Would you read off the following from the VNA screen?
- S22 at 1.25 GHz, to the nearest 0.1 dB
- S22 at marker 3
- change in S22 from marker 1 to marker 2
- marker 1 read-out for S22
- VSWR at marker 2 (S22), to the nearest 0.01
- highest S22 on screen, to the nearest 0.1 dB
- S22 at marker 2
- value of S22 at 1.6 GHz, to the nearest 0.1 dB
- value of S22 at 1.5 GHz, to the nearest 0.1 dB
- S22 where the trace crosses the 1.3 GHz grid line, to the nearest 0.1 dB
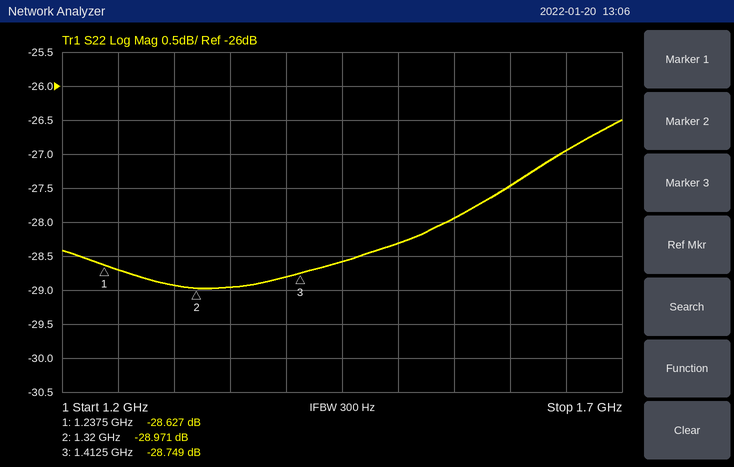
-28.7 dB
-28.749 dB
-0.344 dB
-28.627 dB
1.07
-26.5 dB
-28.971 dB
-27.5 dB
-28.3 dB
-28.9 dB
